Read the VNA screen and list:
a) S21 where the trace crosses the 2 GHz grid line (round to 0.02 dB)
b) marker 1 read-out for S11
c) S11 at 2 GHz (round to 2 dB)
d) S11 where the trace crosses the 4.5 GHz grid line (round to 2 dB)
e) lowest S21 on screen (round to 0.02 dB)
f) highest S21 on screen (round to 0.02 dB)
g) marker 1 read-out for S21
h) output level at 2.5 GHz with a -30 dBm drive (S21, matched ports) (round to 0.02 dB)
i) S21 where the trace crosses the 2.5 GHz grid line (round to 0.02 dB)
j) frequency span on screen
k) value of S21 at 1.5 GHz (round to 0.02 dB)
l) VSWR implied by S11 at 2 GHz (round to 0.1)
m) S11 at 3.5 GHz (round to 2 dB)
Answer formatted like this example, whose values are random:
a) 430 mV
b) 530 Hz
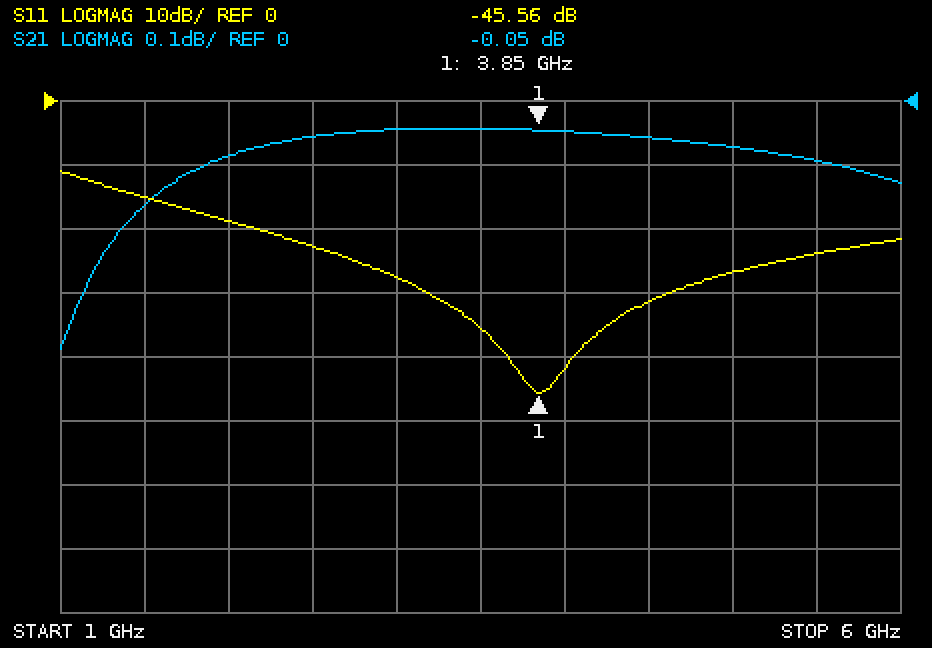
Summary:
a) -0.08 dB
b) -45.56 dB
c) -18 dB
d) -32 dB
e) -0.38 dB
f) -0.04 dB
g) -0.05 dB
h) -30.06 dBm
i) -0.06 dB
j) 5 GHz
k) -0.16 dB
l) 1.3
m) -36 dB
